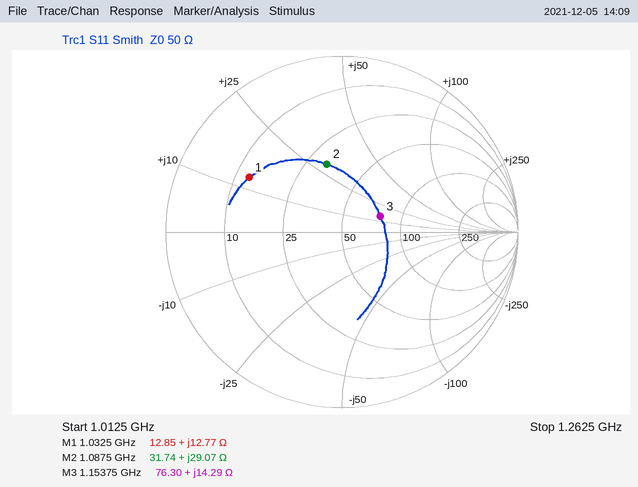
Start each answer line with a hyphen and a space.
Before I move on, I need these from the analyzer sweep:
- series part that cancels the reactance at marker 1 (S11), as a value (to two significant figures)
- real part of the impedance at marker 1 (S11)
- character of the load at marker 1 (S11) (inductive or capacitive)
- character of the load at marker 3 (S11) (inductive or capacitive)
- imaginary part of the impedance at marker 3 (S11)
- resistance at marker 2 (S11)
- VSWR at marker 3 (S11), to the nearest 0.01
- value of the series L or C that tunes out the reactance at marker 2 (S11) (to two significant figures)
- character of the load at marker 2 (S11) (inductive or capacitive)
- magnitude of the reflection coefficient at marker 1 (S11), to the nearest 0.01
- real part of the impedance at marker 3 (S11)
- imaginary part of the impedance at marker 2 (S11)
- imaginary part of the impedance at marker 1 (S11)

- 12 pF
- 12.85 Ω
- inductive
- inductive
- +14.29 Ω
- 31.74 Ω
- 1.62
- 5.0 pF
- inductive
- 0.61
- 76.30 Ω
- +29.07 Ω
- +12.77 Ω
